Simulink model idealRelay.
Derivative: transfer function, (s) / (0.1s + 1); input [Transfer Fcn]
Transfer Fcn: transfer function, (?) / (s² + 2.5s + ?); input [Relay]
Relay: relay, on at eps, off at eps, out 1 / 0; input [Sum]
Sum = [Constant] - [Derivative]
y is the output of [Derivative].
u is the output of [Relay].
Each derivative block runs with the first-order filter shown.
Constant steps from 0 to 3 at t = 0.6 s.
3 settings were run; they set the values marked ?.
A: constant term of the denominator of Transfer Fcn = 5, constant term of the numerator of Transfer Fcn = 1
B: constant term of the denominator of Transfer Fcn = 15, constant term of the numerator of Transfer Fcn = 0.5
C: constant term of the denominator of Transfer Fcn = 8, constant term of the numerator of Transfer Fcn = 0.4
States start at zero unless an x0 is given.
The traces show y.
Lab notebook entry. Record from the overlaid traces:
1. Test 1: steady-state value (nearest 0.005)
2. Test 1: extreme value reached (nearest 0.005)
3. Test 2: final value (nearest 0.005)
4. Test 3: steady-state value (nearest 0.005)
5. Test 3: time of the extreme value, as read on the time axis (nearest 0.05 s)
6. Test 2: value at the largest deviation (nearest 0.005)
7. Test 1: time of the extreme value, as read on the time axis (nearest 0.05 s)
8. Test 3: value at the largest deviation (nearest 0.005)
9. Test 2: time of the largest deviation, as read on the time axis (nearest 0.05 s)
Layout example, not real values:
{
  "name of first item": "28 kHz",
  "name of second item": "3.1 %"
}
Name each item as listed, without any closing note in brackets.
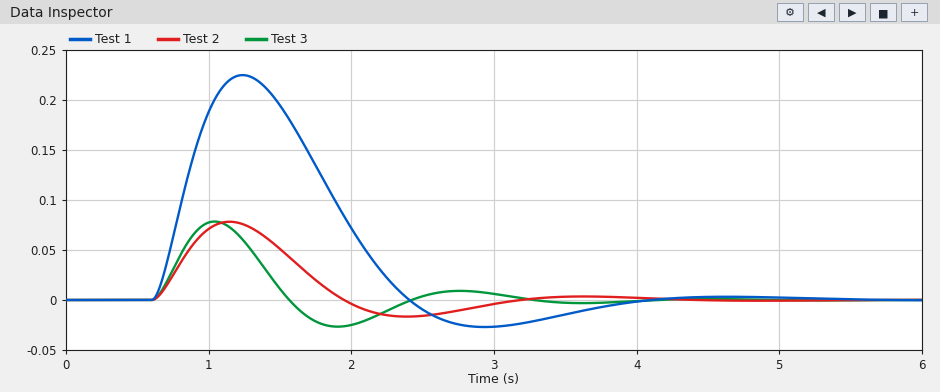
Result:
{
  "Test 1: steady-state value": "0.000",
  "Test 1: extreme value reached": "0.225",
  "Test 2: final value": "0.000",
  "Test 3: steady-state value": "0.000",
  "Test 3: time of the extreme value, as read on the time axis": "1.05 s",
  "Test 2: value at the largest deviation": "0.080",
  "Test 1: time of the extreme value, as read on the time axis": "1.25 s",
  "Test 3: value at the largest deviation": "0.080",
  "Test 2: time of the largest deviation, as read on the time axis": "1.15 s"
}
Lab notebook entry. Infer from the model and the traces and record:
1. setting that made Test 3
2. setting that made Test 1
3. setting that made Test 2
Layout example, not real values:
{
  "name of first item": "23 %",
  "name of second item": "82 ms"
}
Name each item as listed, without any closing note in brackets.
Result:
{
  "setting that made Test 3": "B",
  "setting that made Test 1": "A",
  "setting that made Test 2": "C"
}
